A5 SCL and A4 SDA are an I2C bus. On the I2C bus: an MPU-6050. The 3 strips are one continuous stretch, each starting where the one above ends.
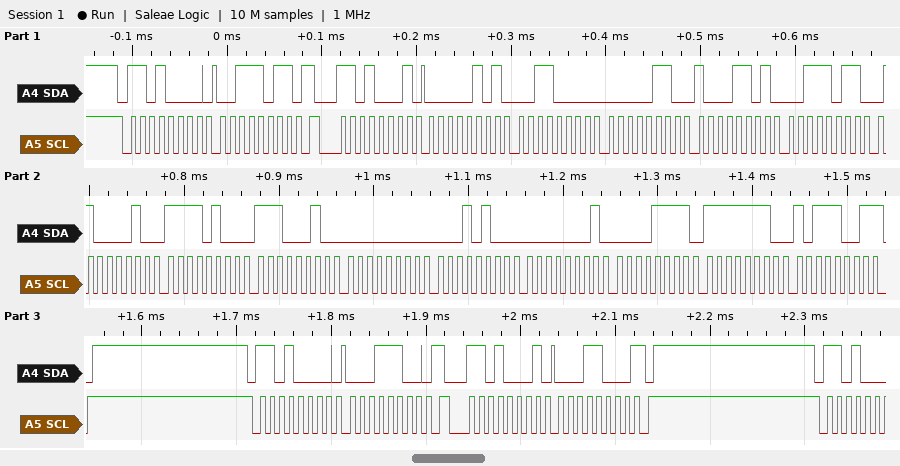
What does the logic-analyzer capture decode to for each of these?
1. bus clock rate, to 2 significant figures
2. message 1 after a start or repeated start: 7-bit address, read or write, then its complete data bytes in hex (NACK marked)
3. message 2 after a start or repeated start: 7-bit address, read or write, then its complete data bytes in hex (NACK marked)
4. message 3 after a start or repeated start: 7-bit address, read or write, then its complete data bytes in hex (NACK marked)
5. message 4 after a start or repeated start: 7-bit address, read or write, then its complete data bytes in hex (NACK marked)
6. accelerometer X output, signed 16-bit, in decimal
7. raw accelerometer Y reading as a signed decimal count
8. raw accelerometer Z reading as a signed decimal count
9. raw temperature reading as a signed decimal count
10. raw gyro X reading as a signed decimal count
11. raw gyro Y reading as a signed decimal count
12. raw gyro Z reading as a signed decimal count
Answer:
100 kHz
0x68 write: 3B
0x68 read: 05 30 06 8D 3B 42 F4 E2 00 14 01 0F FE B9 NACK
0x68 write: 1C
0x68 read: 18 NACK
1328
1677
15170
-2846
20
271
-327
